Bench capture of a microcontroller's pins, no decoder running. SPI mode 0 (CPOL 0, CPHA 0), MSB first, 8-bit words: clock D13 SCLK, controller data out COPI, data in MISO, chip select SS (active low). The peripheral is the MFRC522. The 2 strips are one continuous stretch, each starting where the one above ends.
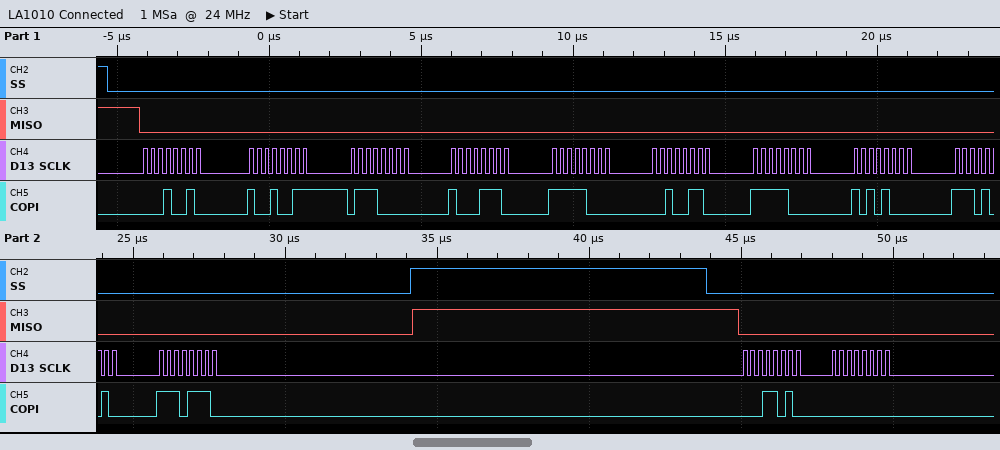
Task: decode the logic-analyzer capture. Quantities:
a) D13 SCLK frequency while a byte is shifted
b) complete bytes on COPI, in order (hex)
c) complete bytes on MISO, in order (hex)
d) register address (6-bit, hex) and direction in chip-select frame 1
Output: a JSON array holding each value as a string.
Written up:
["4 MHz", "12 93 70 8E F8 26 F8 A8 EA EE 1A 00", "00 00 00 00 00 00 00 00 00 00 00 00", "0x09 write"]
